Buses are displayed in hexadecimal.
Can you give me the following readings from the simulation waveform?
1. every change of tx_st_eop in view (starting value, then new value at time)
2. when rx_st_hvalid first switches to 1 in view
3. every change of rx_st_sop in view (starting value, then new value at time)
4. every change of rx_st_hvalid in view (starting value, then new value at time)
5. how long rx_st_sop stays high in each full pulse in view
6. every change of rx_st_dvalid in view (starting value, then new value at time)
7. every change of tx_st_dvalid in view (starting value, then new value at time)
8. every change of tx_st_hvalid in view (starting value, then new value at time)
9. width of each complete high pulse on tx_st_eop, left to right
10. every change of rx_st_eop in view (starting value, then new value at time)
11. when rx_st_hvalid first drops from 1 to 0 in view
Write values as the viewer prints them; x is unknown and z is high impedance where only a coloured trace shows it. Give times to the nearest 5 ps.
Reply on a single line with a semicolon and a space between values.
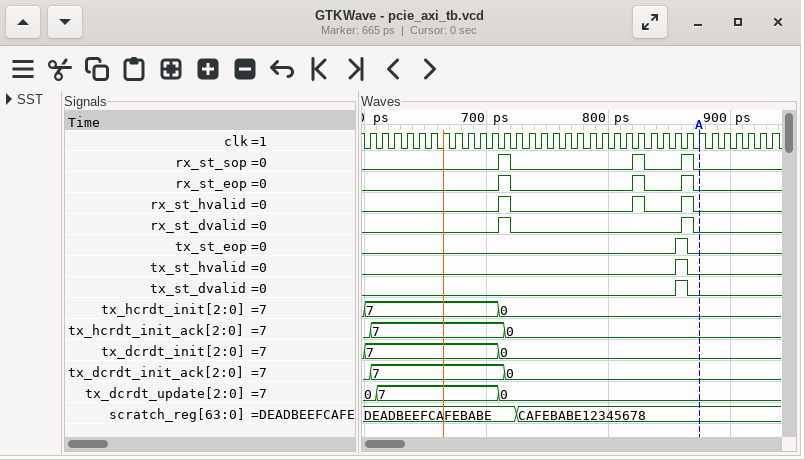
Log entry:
0, 1 at 855 ps, 0 at 865 ps; 710 ps; 0, 1 at 710 ps, 0 at 720 ps, 1 at 820 ps, 0 at 830 ps, 1 at 860 ps, 0 at 870 ps; 0, 1 at 710 ps, 0 at 720 ps, 1 at 820 ps, 0 at 830 ps, 1 at 860 ps, 0 at 870 ps; 10 ps, 10 ps, 10 ps; 0, 1 at 710 ps, 0 at 720 ps, 1 at 860 ps, 0 at 870 ps; 0, 1 at 855 ps, 0 at 865 ps; 0, 1 at 855 ps, 0 at 865 ps; 10 ps; 0, 1 at 710 ps, 0 at 720 ps, 1 at 820 ps, 0 at 830 ps, 1 at 860 ps, 0 at 870 ps; 720 ps
